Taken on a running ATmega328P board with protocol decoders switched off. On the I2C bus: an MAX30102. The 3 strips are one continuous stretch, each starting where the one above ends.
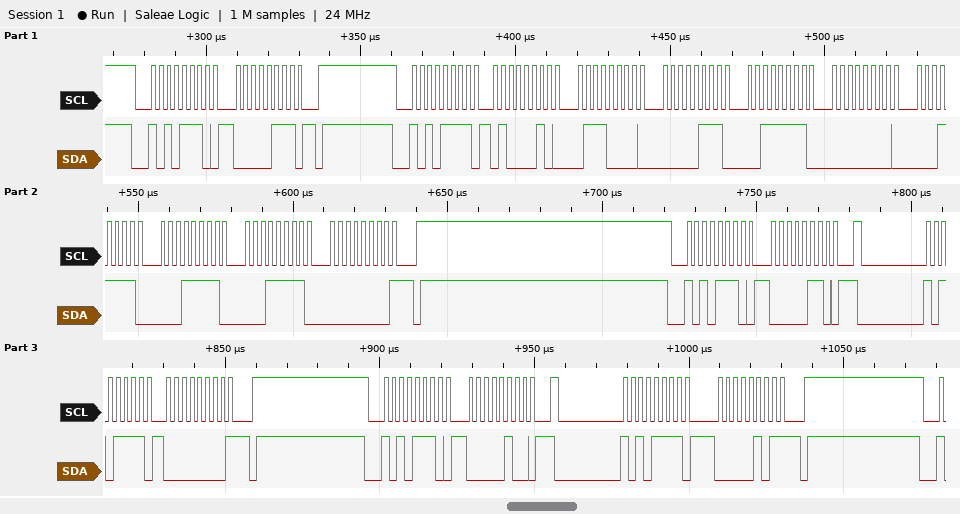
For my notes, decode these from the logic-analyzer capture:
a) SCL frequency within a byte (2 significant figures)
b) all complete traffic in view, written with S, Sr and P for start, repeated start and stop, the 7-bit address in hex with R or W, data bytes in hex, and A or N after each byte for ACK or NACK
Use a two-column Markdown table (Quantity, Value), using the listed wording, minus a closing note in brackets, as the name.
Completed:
| Quantity | Value |
|---|---|
| SCL frequency within a byte | 400 kHz |
| all complete traffic in view, written with S, Sr and P for start, repeated start and stop, the 7-bit address in hex with R or W, data bytes in hex, and A or N after each byte for ACK or NACK | S 57W A 07 A P S 57R A 42 A 70 A 07 A 3F A 00 A 1F A 1F A 1F A 00 N P S 57W A 06 A Sr 57R A 00 N P S 57W A 04 A Sr 57R A 05 N P |
